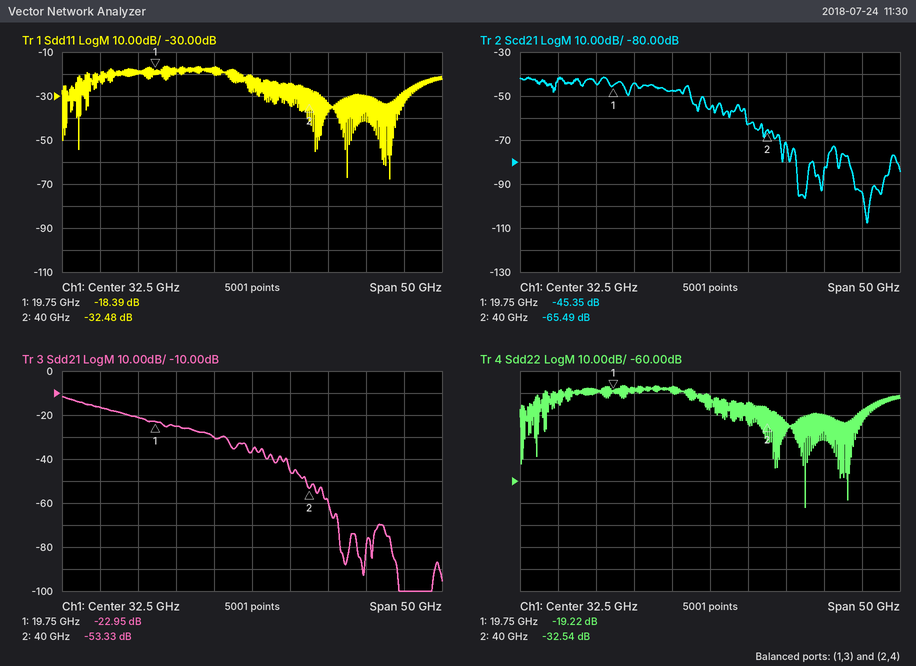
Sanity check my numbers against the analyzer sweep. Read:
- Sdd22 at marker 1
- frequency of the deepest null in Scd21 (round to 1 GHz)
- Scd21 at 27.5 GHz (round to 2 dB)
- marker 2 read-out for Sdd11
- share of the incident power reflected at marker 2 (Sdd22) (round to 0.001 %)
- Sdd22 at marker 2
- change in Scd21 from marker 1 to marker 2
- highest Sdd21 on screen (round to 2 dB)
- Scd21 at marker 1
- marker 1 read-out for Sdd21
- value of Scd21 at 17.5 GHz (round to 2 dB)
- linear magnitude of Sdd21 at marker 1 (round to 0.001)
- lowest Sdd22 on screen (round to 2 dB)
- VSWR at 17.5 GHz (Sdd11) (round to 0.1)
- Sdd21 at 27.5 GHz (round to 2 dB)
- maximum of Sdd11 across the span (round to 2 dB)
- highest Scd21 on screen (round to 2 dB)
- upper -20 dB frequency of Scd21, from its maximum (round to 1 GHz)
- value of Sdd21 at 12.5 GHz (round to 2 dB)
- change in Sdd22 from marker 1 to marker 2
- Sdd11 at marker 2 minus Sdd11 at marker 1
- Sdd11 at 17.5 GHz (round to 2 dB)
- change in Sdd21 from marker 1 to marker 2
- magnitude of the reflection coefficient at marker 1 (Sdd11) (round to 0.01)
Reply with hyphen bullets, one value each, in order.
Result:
- -19.22 dB
- 53 GHz
- -48 dB
- -32.48 dB
- 0.056 %
- -32.54 dB
- -20.14 dB
- -12 dB
- -45.35 dB
- -22.95 dB
- -44 dB
- 0.071
- -72 dB
- 1.2
- -30 dB
- -16 dB
- -42 dB
- 37 GHz
- -16 dB
- -13.32 dB
- -14.09 dB
- -20 dB
- -30.38 dB
- 0.12
